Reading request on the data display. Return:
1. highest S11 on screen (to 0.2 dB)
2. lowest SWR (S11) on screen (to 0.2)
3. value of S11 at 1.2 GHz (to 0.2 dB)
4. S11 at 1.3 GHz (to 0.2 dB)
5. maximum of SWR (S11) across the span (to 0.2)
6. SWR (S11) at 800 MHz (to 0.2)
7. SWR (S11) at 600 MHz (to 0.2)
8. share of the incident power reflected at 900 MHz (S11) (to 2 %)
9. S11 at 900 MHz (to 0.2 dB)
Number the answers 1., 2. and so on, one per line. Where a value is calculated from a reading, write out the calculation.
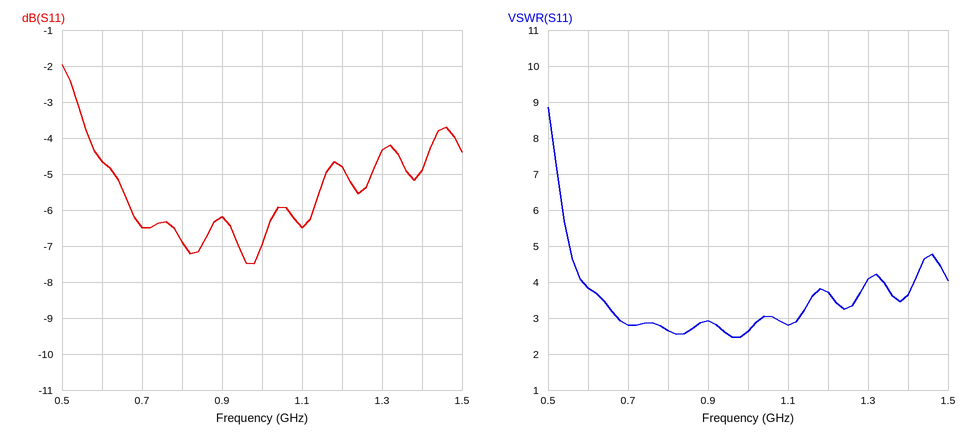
1. -2.0 dB
2. 2.4
3. -4.8 dB
4. -4.4 dB
5. 8.8
6. 2.6
7. 3.8
8. 10^(-6.2/10) ≈ 24 %
9. -6.2 dB
